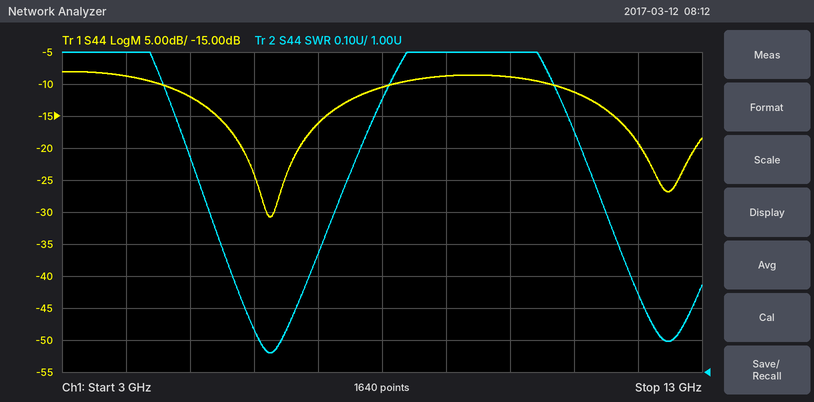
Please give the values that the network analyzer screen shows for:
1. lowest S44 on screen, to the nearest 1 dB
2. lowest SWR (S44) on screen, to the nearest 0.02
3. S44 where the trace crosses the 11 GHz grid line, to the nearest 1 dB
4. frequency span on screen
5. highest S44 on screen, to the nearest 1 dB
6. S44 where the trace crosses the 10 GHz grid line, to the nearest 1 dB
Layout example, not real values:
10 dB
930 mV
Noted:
-31 dB
1.06
-11 dB
10 GHz
-8 dB
-9 dB
